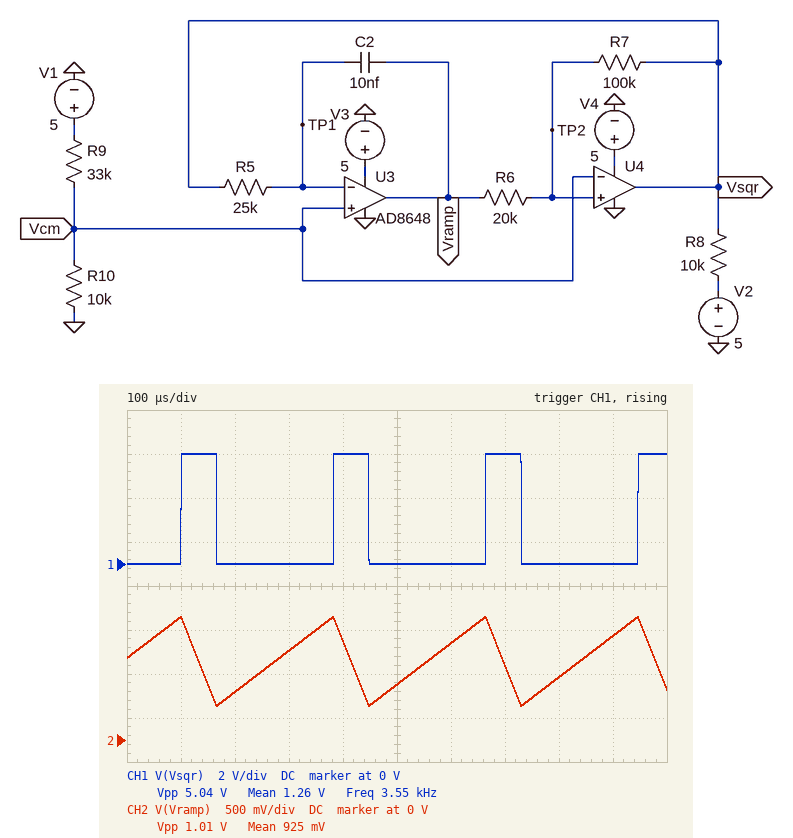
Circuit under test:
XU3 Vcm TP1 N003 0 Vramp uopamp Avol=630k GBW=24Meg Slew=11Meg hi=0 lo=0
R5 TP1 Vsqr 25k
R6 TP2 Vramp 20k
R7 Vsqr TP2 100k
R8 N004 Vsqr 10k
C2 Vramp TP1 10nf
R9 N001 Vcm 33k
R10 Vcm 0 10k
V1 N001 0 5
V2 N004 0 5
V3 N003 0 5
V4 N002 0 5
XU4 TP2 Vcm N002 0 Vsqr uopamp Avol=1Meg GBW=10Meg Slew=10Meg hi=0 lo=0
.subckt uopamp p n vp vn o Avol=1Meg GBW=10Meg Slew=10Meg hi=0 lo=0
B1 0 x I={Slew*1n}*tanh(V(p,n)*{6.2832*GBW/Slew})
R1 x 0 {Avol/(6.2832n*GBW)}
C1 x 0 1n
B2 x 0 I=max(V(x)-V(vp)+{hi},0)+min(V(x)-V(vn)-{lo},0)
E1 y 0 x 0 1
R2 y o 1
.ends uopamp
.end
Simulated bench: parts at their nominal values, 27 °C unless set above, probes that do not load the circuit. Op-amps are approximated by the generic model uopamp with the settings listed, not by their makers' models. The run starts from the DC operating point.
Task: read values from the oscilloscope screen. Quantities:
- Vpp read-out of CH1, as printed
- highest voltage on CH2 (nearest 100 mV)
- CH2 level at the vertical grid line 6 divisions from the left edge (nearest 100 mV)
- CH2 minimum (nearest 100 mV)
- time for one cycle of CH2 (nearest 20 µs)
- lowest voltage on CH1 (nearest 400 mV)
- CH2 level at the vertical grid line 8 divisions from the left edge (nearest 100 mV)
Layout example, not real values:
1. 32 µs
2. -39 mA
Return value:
1. 5.04 V
2. 1.4 V
3. 1.1 V
4. 400 mV
5. 280 µs
6. 0 V
7. 700 mV
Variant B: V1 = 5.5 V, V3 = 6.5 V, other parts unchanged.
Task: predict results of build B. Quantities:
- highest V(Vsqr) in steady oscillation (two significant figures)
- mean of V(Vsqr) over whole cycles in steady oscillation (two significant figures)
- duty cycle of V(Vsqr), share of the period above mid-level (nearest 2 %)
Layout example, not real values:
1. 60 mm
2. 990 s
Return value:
1. 5.0 V
2. 1.3 V
3. 26 %
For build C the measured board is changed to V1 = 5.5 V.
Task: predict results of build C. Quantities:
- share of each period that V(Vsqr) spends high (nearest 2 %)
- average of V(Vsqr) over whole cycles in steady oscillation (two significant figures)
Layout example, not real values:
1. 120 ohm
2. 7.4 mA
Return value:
1. 26 %
2. 1.3 V
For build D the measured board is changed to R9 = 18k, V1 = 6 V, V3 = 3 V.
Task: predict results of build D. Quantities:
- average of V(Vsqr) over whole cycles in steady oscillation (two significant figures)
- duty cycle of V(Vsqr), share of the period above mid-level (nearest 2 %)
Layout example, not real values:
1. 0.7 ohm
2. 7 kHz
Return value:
1. 2.1 V
2. 42 %
